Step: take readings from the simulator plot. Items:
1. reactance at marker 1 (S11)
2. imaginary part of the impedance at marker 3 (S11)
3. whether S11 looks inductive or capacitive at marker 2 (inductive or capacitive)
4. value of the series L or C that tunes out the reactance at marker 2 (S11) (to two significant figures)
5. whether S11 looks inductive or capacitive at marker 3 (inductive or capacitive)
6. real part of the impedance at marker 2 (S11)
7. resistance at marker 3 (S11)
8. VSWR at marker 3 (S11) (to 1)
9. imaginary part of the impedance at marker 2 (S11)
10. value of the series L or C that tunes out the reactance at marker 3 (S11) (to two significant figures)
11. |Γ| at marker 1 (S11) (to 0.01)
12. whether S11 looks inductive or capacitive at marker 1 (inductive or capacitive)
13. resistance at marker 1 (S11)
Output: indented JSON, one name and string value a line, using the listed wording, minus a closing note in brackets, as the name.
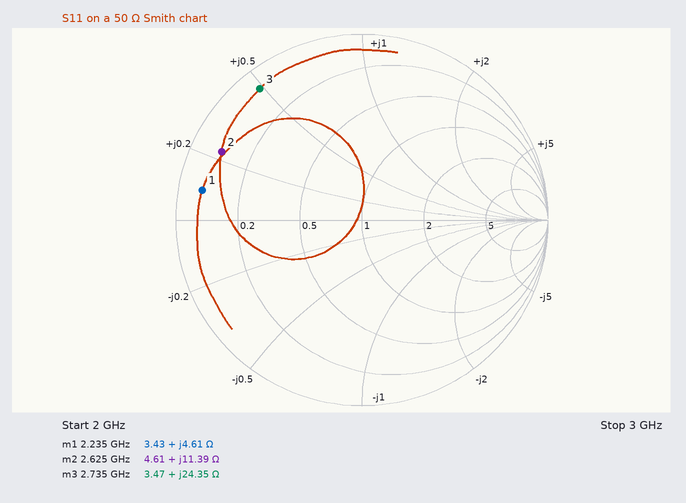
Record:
{
  "reactance at marker 1": "+4.61 Ω",
  "imaginary part of the impedance at marker 3": "+24.35 Ω",
  "whether S11 looks inductive or capacitive at marker 2": "inductive",
  "value of the series L or C that tunes out the reactance at marker 2 (S11)": "5.3 pF",
  "whether S11 looks inductive or capacitive at marker 3": "inductive",
  "real part of the impedance at marker 2": "4.61 Ω",
  "resistance at marker 3": "3.47 Ω",
  "VSWR at marker 3 (S11)": "18",
  "imaginary part of the impedance at marker 2": "+11.39 Ω",
  "value of the series L or C that tunes out the reactance at marker 3 (S11)": "2.4 pF",
  "|Γ| at marker 1 (S11)": "0.87",
  "whether S11 looks inductive or capacitive at marker 1": "inductive",
  "resistance at marker 1": "3.43 Ω"
}
